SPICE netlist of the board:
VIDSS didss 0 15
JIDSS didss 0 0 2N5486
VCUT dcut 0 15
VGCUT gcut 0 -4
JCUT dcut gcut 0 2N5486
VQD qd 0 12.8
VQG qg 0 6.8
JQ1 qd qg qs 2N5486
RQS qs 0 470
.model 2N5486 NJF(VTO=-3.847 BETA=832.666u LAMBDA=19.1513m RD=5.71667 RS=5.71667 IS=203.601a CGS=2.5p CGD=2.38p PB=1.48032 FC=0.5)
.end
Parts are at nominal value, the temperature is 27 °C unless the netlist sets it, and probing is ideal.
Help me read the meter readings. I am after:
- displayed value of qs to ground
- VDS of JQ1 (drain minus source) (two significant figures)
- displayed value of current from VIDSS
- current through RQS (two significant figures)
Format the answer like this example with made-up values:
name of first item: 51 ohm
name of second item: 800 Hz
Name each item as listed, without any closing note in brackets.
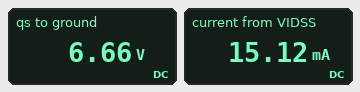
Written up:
displayed value of qs to ground: 6.66 V
VDS of JQ1 (drain minus source): 6.1 V
displayed value of current from VIDSS: 15.12 mA
current through RQS: 14 mA
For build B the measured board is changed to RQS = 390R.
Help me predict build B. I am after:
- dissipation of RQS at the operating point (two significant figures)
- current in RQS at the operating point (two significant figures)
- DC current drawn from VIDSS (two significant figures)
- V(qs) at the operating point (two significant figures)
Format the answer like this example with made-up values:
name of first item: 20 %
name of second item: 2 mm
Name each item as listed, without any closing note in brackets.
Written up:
dissipation of RQS at the operating point: 100 mW
current in RQS at the operating point: 16 mA
DC current drawn from VIDSS: 15 mA
V(qs) at the operating point: 6.4 V
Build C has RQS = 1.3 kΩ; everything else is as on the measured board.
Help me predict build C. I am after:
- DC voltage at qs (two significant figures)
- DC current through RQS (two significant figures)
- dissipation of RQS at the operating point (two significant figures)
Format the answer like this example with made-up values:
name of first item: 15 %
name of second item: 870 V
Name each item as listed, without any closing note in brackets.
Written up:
DC voltage at qs: 8.0 V
DC current through RQS: 6.2 mA
dissipation of RQS at the operating point: 49 mW
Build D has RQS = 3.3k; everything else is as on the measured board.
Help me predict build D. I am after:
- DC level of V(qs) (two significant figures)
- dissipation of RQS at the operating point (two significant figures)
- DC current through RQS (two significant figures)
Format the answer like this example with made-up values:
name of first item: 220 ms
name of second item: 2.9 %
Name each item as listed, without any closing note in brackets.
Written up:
DC level of V(qs): 8.9 V
dissipation of RQS at the operating point: 24 mW
DC current through RQS: 2.7 mA
